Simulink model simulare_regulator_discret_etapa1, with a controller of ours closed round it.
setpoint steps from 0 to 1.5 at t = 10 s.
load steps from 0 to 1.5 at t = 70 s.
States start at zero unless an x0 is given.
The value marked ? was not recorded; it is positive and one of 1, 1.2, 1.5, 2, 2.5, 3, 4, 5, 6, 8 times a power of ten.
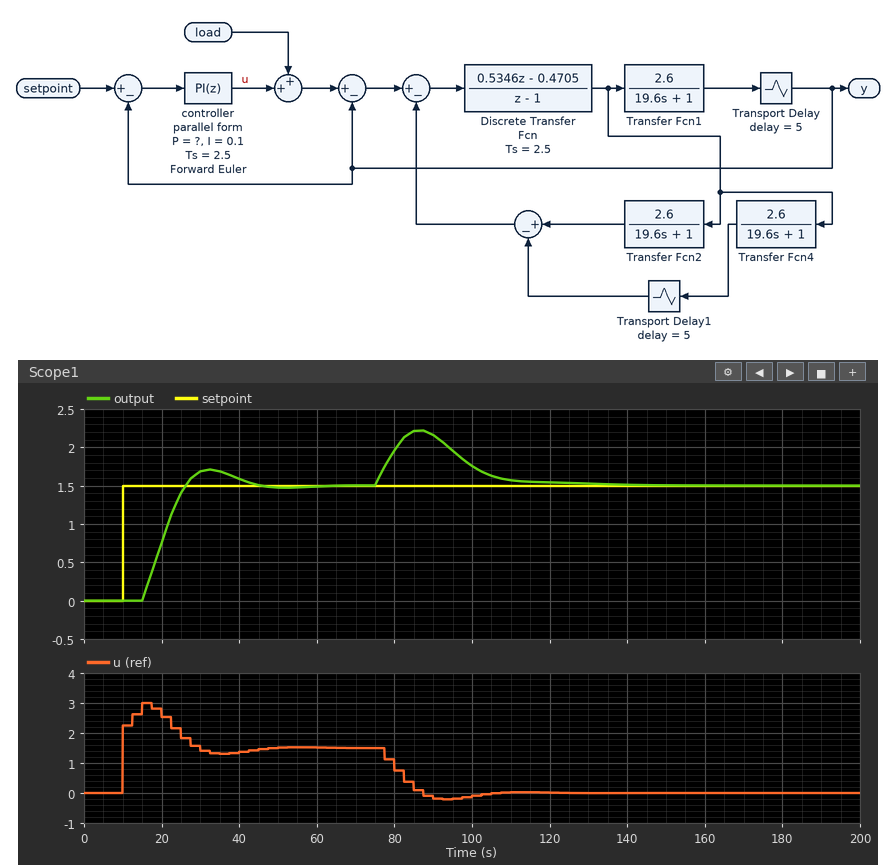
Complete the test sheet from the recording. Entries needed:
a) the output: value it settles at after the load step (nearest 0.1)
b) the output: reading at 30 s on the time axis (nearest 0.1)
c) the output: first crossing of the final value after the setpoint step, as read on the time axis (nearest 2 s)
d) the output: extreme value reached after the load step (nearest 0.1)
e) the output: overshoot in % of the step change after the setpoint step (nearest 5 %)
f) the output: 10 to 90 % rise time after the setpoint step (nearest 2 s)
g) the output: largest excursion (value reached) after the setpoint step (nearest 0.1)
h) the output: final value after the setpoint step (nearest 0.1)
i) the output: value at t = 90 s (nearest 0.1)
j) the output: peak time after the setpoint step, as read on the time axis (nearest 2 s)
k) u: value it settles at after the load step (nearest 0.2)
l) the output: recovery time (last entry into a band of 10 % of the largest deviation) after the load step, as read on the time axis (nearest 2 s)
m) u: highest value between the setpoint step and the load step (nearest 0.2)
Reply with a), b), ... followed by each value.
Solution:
a) 1.5
b) 1.7
c) 26 s
d) 2.2
e) 15 %
f) 8 s
g) 1.7
h) 1.5
i) 2.2
j) 32 s
k) 0.0
l) 110 s
m) 3.0
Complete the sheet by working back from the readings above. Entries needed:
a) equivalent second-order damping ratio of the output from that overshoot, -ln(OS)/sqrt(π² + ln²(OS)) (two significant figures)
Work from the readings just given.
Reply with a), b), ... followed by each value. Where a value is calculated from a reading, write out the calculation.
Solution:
a) ln(0.15) = -1.897; 1.897 / sqrt(9.870 + 3.599) = 0.52
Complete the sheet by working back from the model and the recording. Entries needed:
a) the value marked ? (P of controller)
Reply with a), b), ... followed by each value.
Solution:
a) 1.5
